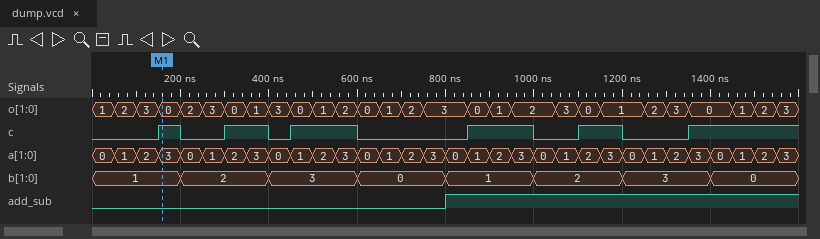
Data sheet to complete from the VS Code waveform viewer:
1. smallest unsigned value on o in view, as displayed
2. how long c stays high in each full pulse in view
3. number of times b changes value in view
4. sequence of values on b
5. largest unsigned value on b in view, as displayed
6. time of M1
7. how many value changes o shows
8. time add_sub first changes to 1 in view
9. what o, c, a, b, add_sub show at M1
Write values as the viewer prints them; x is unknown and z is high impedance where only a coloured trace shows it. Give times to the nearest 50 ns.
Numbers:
0
50 ns, 100 ns, 150 ns, 150 ns, 100 ns
7
1, 2, 3, 0, 1, 2, 3, 0
3
150 ns
27
800 ns
o=0, c=1, a=3, b=1, add_sub=0
